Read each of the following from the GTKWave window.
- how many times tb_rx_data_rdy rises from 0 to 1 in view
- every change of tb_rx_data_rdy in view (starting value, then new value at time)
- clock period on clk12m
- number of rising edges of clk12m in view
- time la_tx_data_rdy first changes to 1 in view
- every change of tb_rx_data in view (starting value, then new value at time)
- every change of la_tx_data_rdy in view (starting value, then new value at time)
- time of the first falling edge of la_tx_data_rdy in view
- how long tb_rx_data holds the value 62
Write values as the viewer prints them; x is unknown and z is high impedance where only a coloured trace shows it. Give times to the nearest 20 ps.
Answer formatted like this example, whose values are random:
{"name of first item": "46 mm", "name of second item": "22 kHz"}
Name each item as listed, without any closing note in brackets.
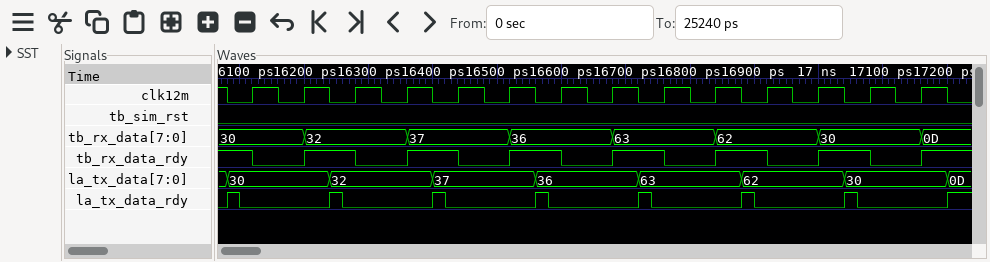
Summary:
{"how many times tb_rx_data_rdy rises from 0 to 1 in view": "7", "every change of tb_rx_data_rdy in view": "1, 0 at 16120 ps, 1 at 16200 ps, 0 at 16280 ps, 1 at 16360 ps, 0 at 16440 ps, 1 at 16520 ps, 0 at 16600 ps, 1 at 16680 ps, 0 at 16760 ps, 1 at 16840 ps, 0 at 16920 ps, 1 at 17000 ps, 0 at 17080 ps, 1 at 17160 ps", "clock period on clk12m": "80 ps", "number of rising edges of clk12m in view": "14", "time la_tx_data_rdy first changes to 1 in view": "16080 ps", "every change of tb_rx_data in view": "30, 32 at 16200 ps, 37 at 16360 ps, 36 at 16520 ps, 63 at 16680 ps, 62 at 16840 ps, 30 at 17000 ps, 0D at 17160 ps", "every change of la_tx_data_rdy in view": "0, 1 at 16080 ps, 0 at 16100 ps, 1 at 16240 ps, 0 at 16260 ps, 1 at 16400 ps, 0 at 16420 ps, 1 at 16560 ps, 0 at 16580 ps, 1 at 16720 ps, 0 at 16740 ps, 1 at 16880 ps, 0 at 16900 ps, 1 at 17040 ps, 0 at 17060 ps, 1 at 17200 ps", "time of the first falling edge of la_tx_data_rdy in view": "16100 ps", "how long tb_rx_data holds the value 62": "160 ps"}
